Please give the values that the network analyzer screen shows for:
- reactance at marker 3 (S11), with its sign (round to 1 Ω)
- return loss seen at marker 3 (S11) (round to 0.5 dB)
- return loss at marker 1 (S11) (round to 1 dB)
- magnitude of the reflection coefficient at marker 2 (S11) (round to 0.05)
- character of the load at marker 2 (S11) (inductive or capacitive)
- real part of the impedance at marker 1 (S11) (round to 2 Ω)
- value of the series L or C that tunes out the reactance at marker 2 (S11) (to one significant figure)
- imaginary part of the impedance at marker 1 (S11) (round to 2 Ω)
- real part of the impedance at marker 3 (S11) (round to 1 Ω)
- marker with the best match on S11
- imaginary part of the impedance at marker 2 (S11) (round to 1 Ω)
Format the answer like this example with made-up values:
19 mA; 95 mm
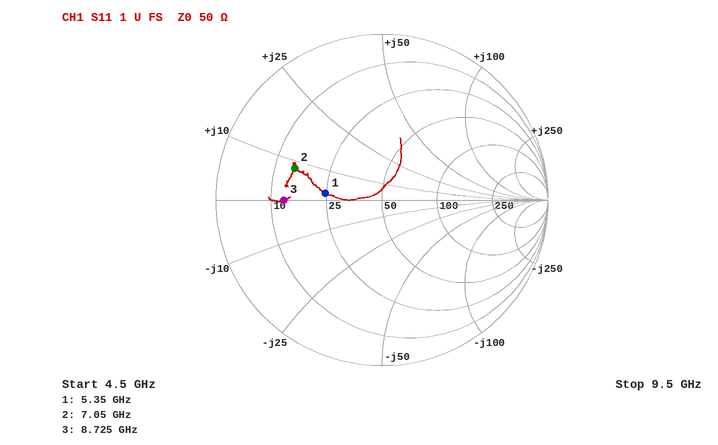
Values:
0 Ω; 4.5 dB; 9 dB; 0.55; inductive; 24 Ω; 3 pF; +2 Ω; 13 Ω; marker 1; +8 Ω
